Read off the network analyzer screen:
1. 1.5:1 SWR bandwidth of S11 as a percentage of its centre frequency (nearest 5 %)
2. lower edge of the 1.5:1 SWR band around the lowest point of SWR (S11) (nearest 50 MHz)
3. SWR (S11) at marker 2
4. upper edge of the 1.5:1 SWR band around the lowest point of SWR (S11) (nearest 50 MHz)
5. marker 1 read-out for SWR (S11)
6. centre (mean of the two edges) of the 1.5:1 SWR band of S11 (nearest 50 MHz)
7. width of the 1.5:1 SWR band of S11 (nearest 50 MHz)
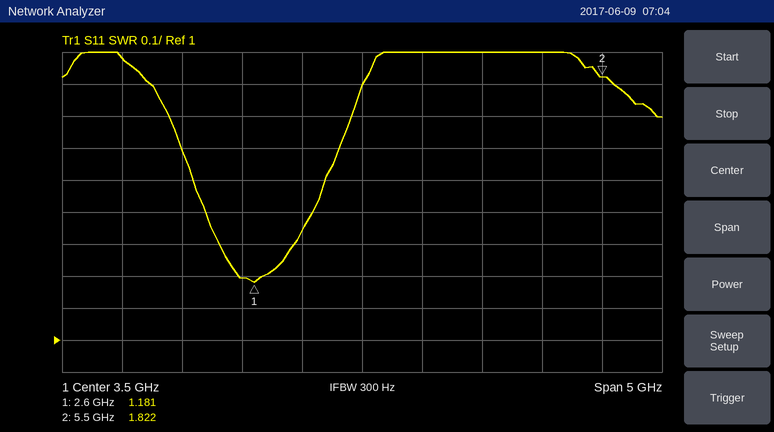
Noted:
40 %
2.10 GHz
1.822
3.20 GHz
1.181
2.65 GHz
1.10 GHz
